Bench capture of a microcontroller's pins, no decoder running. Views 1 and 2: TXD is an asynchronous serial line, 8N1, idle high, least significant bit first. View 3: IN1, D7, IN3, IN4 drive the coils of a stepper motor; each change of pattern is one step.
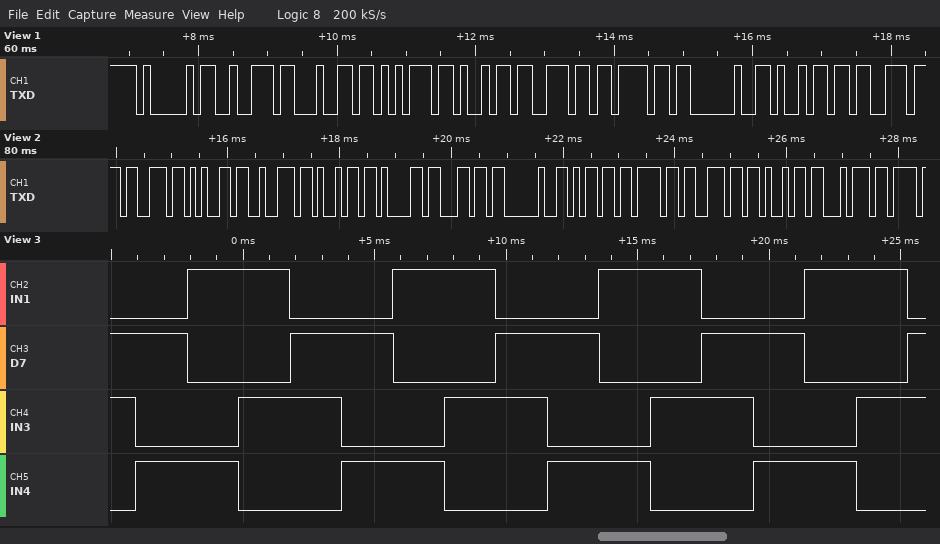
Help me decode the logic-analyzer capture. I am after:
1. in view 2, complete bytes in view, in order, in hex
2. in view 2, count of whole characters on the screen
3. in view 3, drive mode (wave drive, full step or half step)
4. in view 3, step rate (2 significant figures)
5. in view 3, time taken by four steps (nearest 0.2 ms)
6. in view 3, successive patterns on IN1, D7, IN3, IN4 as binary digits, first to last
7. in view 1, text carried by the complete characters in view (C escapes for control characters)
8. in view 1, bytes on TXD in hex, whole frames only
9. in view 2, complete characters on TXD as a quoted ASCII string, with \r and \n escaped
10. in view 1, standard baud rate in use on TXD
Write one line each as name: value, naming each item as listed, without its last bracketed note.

in view 2, complete bytes in view, in order, in hex: 73 65 72 69 61 6C 20 6D 6F 6E 69 74
in view 2, count of whole characters on the screen: 12
in view 3, drive mode: full step
in view 3, step rate: 510 steps/s
in view 3, time taken by four steps: 7.8 ms
in view 3, successive patterns on IN1, D7, IN3, IN4 as binary digits, first to last: 0110 0101 1001 1010 0110 0101 1001 1010 0110 0101 1001 1010 0110 0101 1001 1010 0110
in view 1, text carried by the complete characters in view: "Arduino is"
in view 1, bytes on TXD in hex, whole frames only: 41 72 64 75 69 6E 6F 20 69 73
in view 2, complete characters on TXD as a quoted ASCII string, with \r and \n escaped: "serial monit"
in view 1, standard baud rate in use on TXD: 9600 baud
